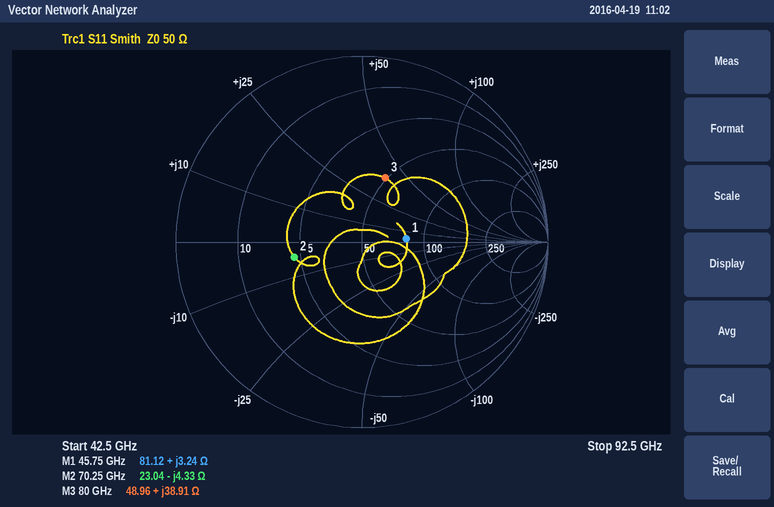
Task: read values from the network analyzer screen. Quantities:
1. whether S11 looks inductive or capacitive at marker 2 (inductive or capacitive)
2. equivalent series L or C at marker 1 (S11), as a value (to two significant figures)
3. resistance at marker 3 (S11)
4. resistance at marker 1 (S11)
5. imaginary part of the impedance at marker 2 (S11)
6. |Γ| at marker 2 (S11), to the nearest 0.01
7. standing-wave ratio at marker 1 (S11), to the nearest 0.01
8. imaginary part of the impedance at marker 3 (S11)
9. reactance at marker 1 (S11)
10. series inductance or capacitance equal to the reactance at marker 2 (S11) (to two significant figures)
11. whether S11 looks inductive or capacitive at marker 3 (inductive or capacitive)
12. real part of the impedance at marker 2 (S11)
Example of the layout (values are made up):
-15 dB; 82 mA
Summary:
capacitive; 11 pH; 48.96 Ω; 81.12 Ω; -4.33 Ω; 0.37; 1.63; +38.91 Ω; +3.24 Ω; 520 fF; inductive; 23.04 Ω
